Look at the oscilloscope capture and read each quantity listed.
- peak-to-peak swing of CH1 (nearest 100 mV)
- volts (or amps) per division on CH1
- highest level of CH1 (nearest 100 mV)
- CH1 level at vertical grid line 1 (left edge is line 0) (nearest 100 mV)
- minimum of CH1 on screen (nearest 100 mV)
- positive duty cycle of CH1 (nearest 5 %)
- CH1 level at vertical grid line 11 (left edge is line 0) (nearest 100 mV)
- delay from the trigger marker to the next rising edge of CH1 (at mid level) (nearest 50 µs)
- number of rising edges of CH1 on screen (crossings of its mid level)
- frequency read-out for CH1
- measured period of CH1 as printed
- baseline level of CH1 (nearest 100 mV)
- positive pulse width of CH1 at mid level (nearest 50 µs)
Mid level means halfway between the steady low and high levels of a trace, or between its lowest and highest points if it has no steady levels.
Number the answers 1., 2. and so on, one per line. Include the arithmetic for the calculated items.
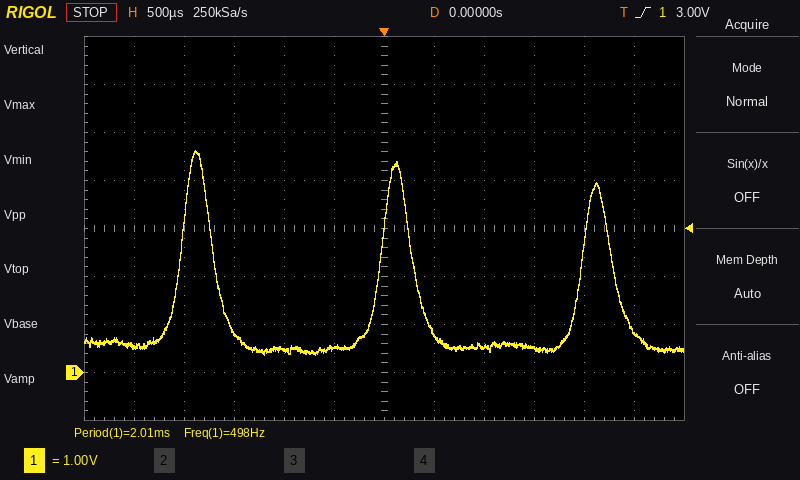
1. 4.6 V − (400 mV) = 4.2 V
2. 1 V
3. 4.6 V
4. 600 mV
5. 400 mV
6. 15 %
7. 900 mV
8. 2.00 ms
9. 3
10. 498 Hz
11. 2.01 ms
12. 600 mV
13. 300 µs
